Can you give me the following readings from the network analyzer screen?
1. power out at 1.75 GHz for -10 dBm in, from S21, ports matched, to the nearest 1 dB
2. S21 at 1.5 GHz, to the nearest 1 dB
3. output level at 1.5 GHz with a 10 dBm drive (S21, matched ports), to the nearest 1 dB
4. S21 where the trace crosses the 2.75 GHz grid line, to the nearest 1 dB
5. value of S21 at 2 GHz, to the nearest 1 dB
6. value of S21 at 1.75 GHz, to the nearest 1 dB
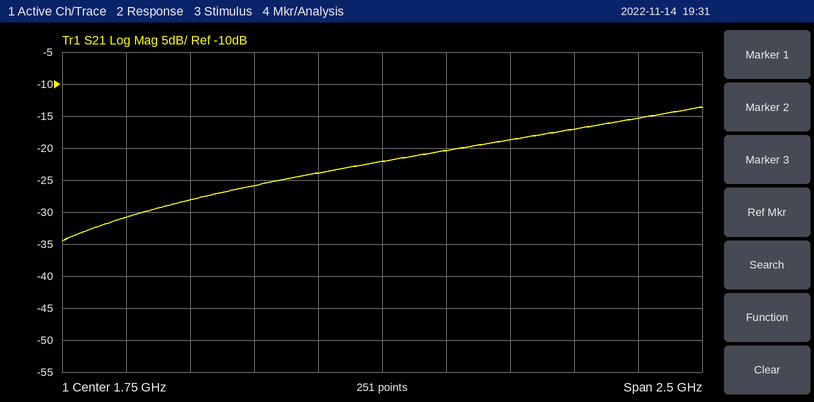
-32 dBm
-24 dB
-14 dBm
-15 dB
-20 dB
-22 dB
